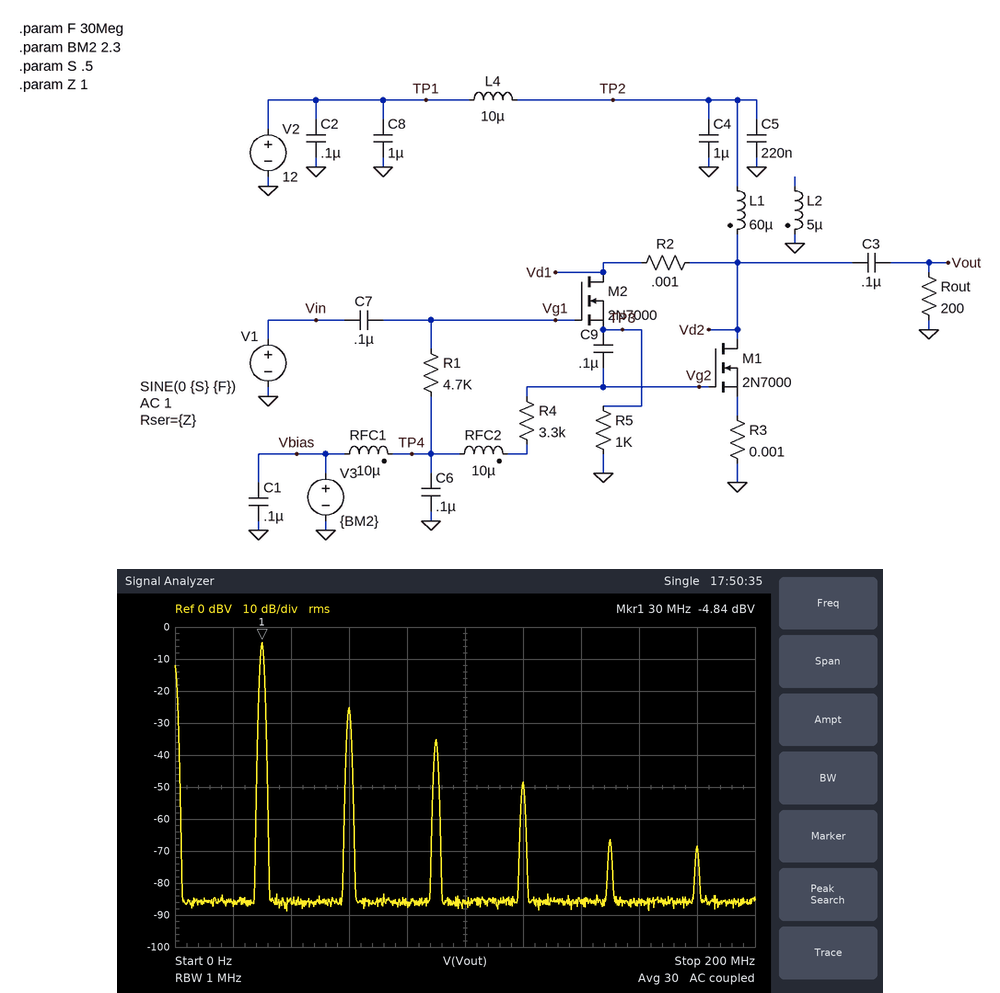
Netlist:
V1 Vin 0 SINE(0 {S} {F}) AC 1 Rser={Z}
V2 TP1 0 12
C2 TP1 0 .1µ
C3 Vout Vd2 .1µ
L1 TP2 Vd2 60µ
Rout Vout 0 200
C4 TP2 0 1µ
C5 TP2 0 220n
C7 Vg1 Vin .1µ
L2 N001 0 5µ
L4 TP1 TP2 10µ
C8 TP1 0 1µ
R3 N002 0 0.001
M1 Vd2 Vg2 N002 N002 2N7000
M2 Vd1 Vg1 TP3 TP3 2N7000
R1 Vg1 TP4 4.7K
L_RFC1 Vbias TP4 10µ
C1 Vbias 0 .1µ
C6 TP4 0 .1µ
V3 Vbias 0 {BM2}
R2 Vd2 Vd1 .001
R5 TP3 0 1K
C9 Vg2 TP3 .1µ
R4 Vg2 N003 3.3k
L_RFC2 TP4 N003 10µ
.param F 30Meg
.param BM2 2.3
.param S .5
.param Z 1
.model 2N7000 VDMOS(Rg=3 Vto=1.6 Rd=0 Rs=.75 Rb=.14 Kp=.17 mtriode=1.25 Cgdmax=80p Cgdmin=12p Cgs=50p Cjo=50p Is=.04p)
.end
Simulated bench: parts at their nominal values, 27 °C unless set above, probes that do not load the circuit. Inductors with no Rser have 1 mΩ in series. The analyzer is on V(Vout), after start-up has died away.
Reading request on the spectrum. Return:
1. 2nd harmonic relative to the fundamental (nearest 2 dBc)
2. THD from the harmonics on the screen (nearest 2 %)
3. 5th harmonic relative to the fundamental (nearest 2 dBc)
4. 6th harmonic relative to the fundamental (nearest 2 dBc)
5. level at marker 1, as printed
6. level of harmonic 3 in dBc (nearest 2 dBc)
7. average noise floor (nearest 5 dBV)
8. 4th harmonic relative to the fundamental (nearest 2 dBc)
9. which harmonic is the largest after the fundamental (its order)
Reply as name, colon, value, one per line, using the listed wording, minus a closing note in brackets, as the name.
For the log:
2nd harmonic relative to the fundamental: -20 dBc
THD from the harmonics on the screen: 10 %
5th harmonic relative to the fundamental: -62 dBc
6th harmonic relative to the fundamental: -64 dBc
level at marker 1, as printed: -4.84 dBV
level of harmonic 3 in dBc: -30 dBc
average noise floor: -85 dBV
4th harmonic relative to the fundamental: -44 dBc
which harmonic is the largest after the fundamental: 2
